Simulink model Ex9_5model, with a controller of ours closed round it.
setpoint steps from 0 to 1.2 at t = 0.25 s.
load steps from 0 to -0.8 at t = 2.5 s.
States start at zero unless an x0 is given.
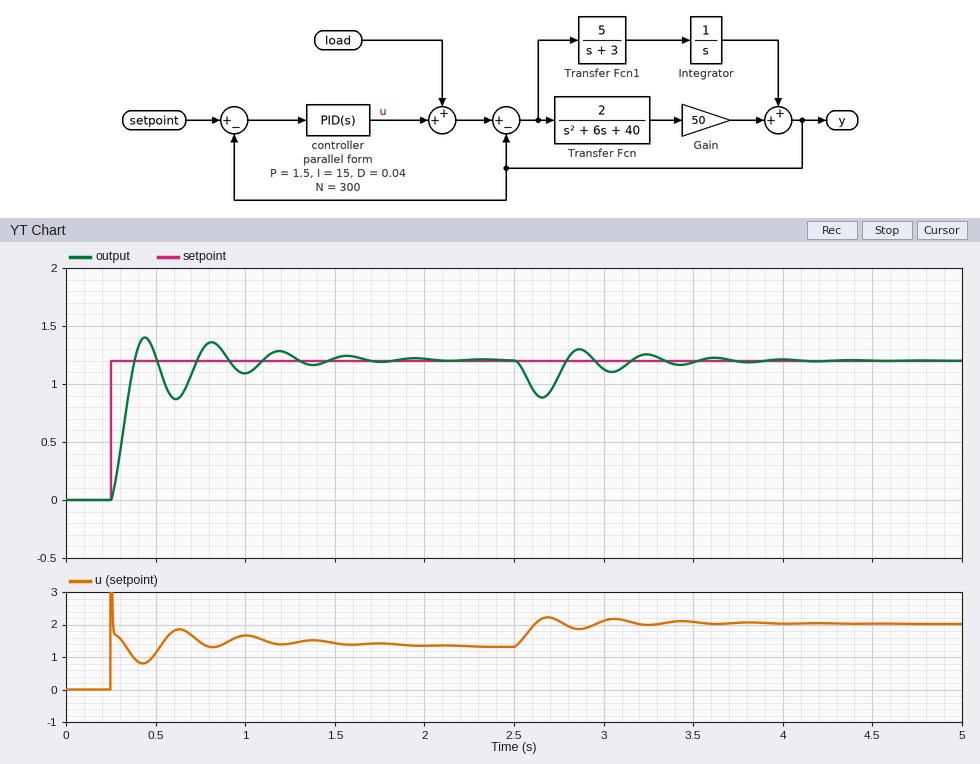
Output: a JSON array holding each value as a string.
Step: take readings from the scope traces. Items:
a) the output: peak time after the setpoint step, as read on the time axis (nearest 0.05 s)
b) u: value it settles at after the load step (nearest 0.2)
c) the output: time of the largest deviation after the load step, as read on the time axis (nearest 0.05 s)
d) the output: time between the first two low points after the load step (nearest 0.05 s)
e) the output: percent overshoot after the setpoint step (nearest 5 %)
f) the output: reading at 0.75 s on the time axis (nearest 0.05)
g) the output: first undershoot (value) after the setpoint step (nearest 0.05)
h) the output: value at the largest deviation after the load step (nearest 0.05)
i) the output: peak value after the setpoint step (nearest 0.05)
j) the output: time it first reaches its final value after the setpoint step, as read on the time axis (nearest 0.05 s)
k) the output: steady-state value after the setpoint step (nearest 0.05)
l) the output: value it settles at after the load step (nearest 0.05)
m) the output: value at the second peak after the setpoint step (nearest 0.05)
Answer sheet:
["0.45 s", "2.0", "2.65 s", "0.40 s", "15 %", "1.25", "0.85", "0.90", "1.40", "0.40 s", "1.20", "1.20", "1.35"]
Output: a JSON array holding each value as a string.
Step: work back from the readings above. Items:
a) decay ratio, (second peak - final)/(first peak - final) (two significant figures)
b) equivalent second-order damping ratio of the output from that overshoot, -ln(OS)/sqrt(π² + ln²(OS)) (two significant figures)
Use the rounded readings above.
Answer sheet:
["0.75", "0.52"]
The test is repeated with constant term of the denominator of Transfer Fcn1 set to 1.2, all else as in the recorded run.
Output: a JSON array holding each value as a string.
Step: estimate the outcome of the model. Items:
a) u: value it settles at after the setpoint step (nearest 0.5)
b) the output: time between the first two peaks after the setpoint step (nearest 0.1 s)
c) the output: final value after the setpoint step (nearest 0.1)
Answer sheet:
["1.0", "0.4 s", "1.2"]
